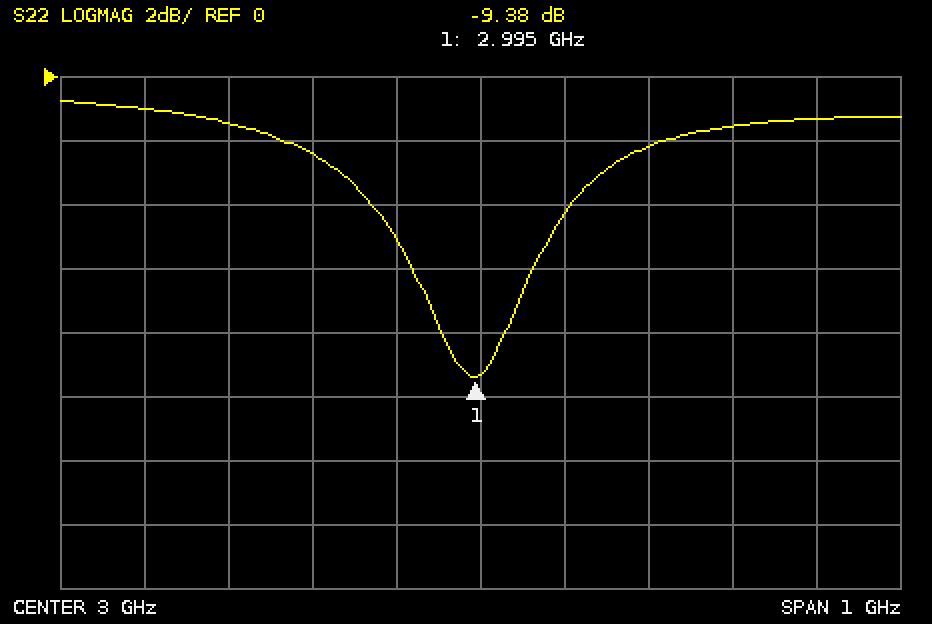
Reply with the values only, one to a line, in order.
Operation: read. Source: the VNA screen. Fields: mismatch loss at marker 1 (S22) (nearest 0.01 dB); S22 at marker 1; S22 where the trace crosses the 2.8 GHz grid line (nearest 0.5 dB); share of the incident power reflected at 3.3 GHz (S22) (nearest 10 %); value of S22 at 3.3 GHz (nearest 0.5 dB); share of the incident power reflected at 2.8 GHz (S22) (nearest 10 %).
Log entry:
0.53 dB
-9.38 dB
-2.5 dB
70 %
-1.5 dB
60 %
